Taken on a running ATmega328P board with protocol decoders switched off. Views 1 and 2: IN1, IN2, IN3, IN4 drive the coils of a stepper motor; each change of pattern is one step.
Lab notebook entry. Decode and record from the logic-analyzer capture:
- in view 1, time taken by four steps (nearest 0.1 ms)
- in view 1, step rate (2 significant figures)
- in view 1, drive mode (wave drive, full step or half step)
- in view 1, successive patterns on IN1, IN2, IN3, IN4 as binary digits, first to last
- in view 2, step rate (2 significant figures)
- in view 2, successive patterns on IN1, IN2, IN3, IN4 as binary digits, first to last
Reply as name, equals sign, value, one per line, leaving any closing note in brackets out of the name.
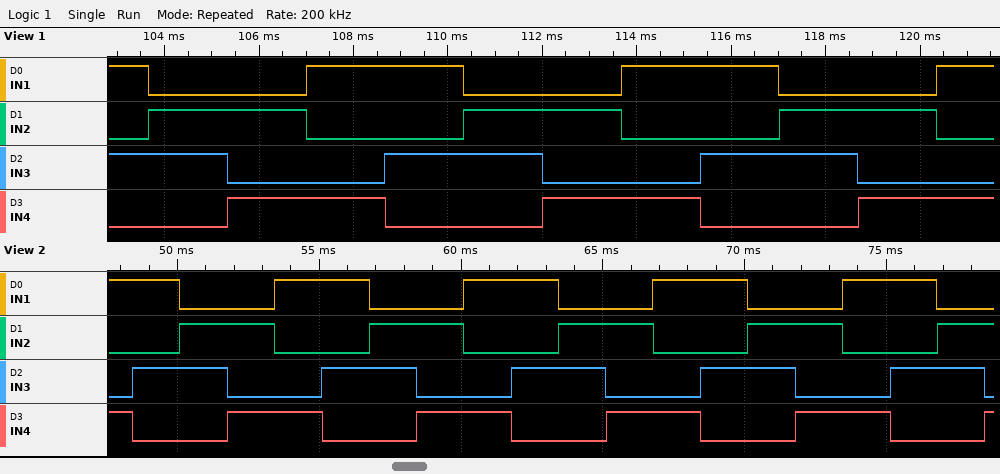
in view 1, time taken by four steps = 6.7 ms
in view 1, step rate = 600 steps/s
in view 1, drive mode = full step
in view 1, successive patterns on IN1, IN2, IN3, IN4 as binary digits, first to last = 1010 0110 0101 1001 1010 0110 0101 1001 1010 0110 0101 1001
in view 2, step rate = 600 steps/s
in view 2, successive patterns on IN1, IN2, IN3, IN4 as binary digits, first to last = 1001 1010 0110 0101 1001 1010 0110 0101 1001 1010 0110 0101 1001 1010 0110 0101 1001 1010 0110 0101
